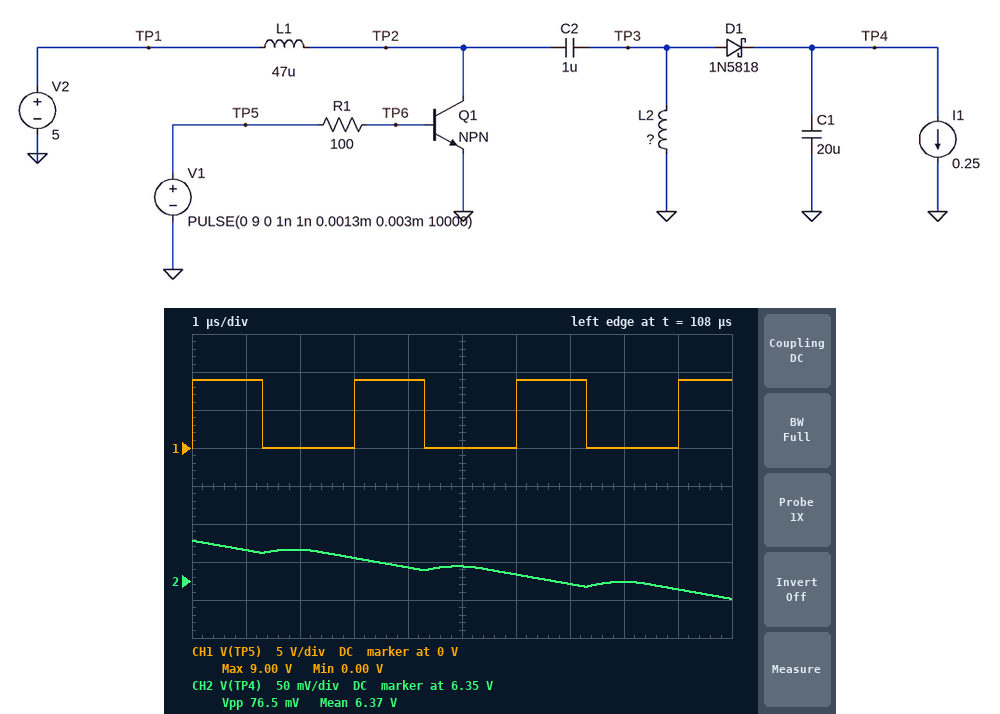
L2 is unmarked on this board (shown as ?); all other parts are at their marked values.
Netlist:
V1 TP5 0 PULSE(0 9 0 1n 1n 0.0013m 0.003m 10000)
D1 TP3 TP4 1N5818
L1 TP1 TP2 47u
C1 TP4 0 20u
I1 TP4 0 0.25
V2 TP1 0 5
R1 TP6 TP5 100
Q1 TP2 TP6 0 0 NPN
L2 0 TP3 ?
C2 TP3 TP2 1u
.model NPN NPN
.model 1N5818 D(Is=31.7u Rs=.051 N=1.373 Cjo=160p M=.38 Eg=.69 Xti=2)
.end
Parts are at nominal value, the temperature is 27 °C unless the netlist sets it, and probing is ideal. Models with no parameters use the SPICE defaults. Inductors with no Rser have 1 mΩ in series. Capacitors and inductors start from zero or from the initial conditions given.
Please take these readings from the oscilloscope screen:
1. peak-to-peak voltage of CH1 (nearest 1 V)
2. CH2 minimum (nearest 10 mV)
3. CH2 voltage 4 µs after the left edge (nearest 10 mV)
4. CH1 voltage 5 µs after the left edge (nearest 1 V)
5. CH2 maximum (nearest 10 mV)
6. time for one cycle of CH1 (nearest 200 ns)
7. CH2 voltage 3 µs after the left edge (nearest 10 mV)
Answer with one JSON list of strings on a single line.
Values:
["9 V", "6.33 V", "6.37 V", "0 V", "6.40 V", "3.0 µs", "6.38 V"]
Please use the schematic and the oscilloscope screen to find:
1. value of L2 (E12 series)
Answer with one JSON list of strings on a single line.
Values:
["18 µH"]
